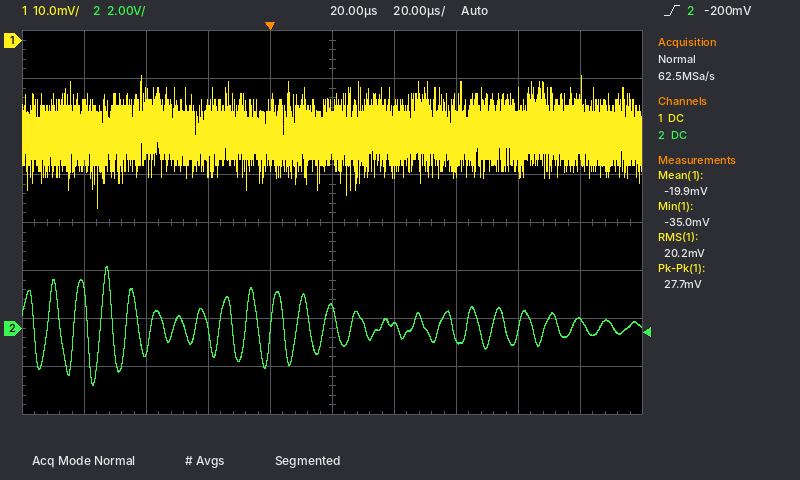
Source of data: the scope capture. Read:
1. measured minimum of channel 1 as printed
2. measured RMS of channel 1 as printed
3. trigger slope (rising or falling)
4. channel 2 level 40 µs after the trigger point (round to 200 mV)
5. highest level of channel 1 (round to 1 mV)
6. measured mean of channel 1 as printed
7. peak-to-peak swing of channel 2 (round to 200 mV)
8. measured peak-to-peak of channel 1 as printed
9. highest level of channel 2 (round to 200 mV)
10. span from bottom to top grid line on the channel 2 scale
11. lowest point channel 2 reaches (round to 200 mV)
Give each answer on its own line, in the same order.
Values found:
-35.0 mV
20.2 mV
rising
200 mV
-7 mV
-19.9 mV
5.0 V
27.7 mV
2.6 V
16 V
-2.4 V
